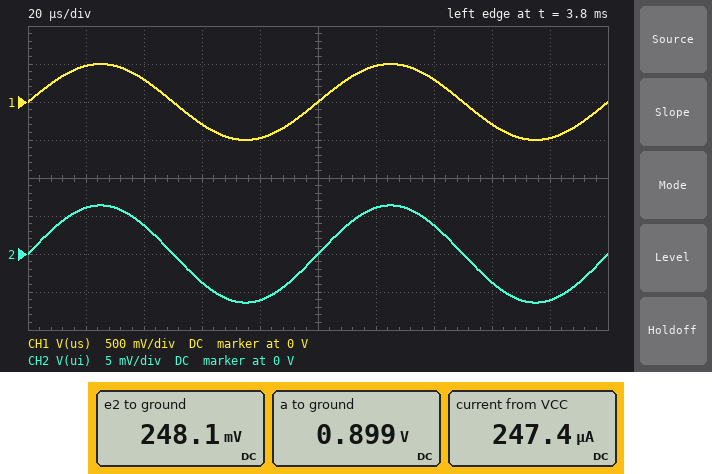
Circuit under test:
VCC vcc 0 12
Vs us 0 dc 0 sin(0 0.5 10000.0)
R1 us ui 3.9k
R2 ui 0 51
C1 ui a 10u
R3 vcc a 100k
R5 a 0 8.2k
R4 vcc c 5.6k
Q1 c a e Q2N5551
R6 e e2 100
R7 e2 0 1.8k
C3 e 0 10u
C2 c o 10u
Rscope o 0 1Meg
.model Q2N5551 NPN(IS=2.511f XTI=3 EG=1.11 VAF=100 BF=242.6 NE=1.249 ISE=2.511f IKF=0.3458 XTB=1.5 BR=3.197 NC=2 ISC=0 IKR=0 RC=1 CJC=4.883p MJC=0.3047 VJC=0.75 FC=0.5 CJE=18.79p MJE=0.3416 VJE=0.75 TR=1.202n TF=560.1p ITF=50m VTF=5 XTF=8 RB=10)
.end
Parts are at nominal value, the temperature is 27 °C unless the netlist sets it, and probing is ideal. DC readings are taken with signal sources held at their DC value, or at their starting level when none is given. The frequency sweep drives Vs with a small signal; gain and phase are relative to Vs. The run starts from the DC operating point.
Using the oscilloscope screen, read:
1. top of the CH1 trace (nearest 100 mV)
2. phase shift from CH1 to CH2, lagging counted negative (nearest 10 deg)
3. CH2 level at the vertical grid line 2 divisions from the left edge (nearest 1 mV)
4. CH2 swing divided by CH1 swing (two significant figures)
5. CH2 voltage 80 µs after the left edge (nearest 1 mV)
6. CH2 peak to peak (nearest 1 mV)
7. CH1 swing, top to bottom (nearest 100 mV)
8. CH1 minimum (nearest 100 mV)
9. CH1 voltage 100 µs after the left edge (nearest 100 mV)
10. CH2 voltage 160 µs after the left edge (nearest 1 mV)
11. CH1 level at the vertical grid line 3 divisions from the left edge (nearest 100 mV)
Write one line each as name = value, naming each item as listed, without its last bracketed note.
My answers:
top of the CH1 trace = 500 mV
phase shift from CH1 to CH2, lagging counted negative = 0 deg
CH2 level at the vertical grid line 2 divisions from the left edge = 4 mV
CH2 swing divided by CH1 swing = 0.013
CH2 voltage 80 µs after the left edge = -6 mV
CH2 peak to peak = 13 mV
CH1 swing, top to bottom = 1.0 V
CH1 minimum = -500 mV
CH1 voltage 100 µs after the left edge = 0 V
CH2 voltage 160 µs after the left edge = -4 mV
CH1 level at the vertical grid line 3 divisions from the left edge = -300 mV
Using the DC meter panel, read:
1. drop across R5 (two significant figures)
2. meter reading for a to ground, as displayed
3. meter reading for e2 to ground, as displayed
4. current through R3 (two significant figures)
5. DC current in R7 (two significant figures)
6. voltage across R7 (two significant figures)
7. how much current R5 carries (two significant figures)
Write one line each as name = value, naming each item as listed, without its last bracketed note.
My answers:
drop across R5 = 900 mV
meter reading for a to ground, as displayed = 0.899 V
meter reading for e2 to ground, as displayed = 248.1 mV
current through R3 = 110 µA
DC current in R7 = 140 µA
voltage across R7 = 250 mV
how much current R5 carries = 110 µA
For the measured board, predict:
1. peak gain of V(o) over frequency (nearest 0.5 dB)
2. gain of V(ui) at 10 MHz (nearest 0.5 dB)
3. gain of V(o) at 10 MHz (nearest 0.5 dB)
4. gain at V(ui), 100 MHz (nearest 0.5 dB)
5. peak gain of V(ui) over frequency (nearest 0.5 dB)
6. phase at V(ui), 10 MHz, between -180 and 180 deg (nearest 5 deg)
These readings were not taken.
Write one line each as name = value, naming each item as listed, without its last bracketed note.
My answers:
peak gain of V(o) over frequency = -8.5 dB
gain of V(ui) at 10 MHz = -39.0 dB
gain of V(o) at 10 MHz = -11.5 dB
gain at V(ui), 100 MHz = -42.5 dB
peak gain of V(ui) over frequency = -38.0 dB
phase at V(ui), 10 MHz, between -180 and 180 deg = -10 deg
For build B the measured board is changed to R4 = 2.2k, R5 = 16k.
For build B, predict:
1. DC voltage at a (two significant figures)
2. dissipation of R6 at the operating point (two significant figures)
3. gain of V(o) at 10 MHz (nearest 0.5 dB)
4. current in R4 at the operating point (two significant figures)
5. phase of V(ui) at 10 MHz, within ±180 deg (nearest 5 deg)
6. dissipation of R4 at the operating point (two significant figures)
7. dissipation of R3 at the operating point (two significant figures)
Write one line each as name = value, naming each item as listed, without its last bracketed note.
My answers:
DC voltage at a = 1.6 V
dissipation of R6 at the operating point = 24 µW
gain of V(o) at 10 MHz = -7.5 dB
current in R4 at the operating point = 480 µA
phase of V(ui) at 10 MHz, within ±180 deg = -20 deg
dissipation of R4 at the operating point = 510 µW
dissipation of R3 at the operating point = 1.1 mW
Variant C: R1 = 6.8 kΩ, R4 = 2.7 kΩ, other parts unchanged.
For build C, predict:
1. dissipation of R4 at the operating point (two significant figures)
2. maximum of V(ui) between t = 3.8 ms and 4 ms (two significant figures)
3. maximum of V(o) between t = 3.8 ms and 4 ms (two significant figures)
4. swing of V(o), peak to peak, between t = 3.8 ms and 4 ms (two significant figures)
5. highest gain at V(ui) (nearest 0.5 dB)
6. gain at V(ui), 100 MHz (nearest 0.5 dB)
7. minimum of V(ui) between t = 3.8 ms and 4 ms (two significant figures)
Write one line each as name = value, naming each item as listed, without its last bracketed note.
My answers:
dissipation of R4 at the operating point = 50 µW
maximum of V(ui) between t = 3.8 ms and 4 ms = 3.7 mV
maximum of V(o) between t = 3.8 ms and 4 ms = 50 mV
swing of V(o), peak to peak, between t = 3.8 ms and 4 ms = 100 mV
highest gain at V(ui) = -42.5 dB
gain at V(ui), 100 MHz = -47.5 dB
minimum of V(ui) between t = 3.8 ms and 4 ms = -3.7 mV
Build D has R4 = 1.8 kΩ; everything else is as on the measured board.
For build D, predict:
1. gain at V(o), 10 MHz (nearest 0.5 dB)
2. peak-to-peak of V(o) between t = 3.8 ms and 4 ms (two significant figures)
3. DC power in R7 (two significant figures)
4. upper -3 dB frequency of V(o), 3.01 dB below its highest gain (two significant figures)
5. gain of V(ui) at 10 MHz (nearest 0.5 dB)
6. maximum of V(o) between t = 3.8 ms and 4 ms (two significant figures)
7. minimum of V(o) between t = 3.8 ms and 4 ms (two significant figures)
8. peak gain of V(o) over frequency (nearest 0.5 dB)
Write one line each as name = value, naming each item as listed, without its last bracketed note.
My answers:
gain at V(o), 10 MHz = -19.0 dB
peak-to-peak of V(o) between t = 3.8 ms and 4 ms = 120 mV
DC power in R7 = 34 µW
upper -3 dB frequency of V(o), 3.01 dB below its highest gain = 26 MHz
gain of V(ui) at 10 MHz = -38.0 dB
maximum of V(o) between t = 3.8 ms and 4 ms = 56 mV
minimum of V(o) between t = 3.8 ms and 4 ms = -65 mV
peak gain of V(o) over frequency = -18.5 dB
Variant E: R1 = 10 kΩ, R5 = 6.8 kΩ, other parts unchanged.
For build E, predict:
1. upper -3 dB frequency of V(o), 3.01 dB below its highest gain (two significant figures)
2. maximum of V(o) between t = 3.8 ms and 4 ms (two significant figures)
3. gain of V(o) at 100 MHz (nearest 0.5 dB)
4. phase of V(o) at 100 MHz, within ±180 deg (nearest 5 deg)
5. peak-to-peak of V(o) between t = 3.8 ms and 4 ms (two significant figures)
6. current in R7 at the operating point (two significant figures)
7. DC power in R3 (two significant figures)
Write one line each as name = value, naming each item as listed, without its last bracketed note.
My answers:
upper -3 dB frequency of V(o), 3.01 dB below its highest gain = 11 MHz
maximum of V(o) between t = 3.8 ms and 4 ms = 38 mV
gain of V(o) at 100 MHz = -43.0 dB
phase of V(o) at 100 MHz, within ±180 deg = 25 deg
peak-to-peak of V(o) between t = 3.8 ms and 4 ms = 78 mV
current in R7 at the operating point = 73 µA
DC power in R3 = 1.3 mW
